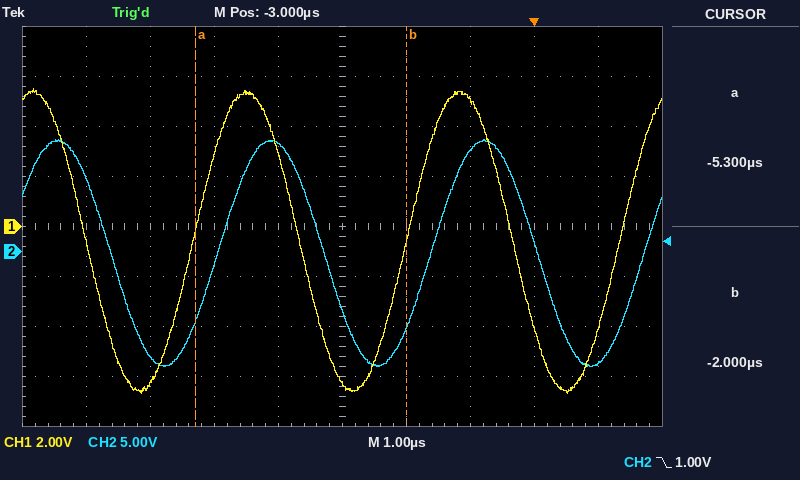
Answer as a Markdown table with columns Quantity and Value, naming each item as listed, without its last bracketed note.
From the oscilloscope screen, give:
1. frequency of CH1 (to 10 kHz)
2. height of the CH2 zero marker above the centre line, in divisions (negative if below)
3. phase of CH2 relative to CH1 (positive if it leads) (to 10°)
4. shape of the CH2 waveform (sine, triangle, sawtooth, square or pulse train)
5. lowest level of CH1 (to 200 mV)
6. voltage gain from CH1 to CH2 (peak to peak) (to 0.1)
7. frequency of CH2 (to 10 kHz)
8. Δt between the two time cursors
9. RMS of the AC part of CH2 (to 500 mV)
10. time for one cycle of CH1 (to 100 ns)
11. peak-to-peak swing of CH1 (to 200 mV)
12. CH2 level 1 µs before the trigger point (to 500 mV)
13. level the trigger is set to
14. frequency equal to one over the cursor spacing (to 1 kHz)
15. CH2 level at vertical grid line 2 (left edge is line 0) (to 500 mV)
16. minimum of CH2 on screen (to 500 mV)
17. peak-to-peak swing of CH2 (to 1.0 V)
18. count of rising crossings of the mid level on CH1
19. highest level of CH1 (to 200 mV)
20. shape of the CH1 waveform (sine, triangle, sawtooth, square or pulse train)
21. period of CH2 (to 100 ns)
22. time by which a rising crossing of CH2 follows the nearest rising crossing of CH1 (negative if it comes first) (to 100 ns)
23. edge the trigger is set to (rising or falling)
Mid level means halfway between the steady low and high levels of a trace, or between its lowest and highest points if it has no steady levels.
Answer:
| Quantity | Value |
|---|---|
| frequency of CH1 | 300 kHz |
| height of the CH2 zero marker above the centre line, in divisions | -0.5 div |
| phase of CH2 relative to CH1 (positive if it leads) | -40° |
| shape of the CH2 waveform | sine |
| lowest level of CH1 | -6.6 V |
| voltage gain from CH1 to CH2 (peak to peak) | 1.9 |
| frequency of CH2 | 300 kHz |
| Δt between the two time cursors | 3.3 µs |
| RMS of the AC part of CH2 | 8.0 V |
| time for one cycle of CH1 | 3.3 µs |
| peak-to-peak swing of CH1 | 12.2 V |
| CH2 level 1 µs before the trigger point | 10.0 V |
| level the trigger is set to | 1.00 V |
| frequency equal to one over the cursor spacing | 303 kHz |
| CH2 level at vertical grid line 2 (left edge is line 0) | -10.5 V |
| minimum of CH2 on screen | -11.5 V |
| peak-to-peak swing of CH2 | 23.0 V |
| count of rising crossings of the mid level on CH1 | 3 |
| highest level of CH1 | 5.6 V |
| shape of the CH1 waveform | sine |
| period of CH2 | 3.3 µs |
| time by which a rising crossing of CH2 follows the nearest rising crossing of CH1 (negative if it comes first) | +400 ns |
| edge the trigger is set to | falling |
